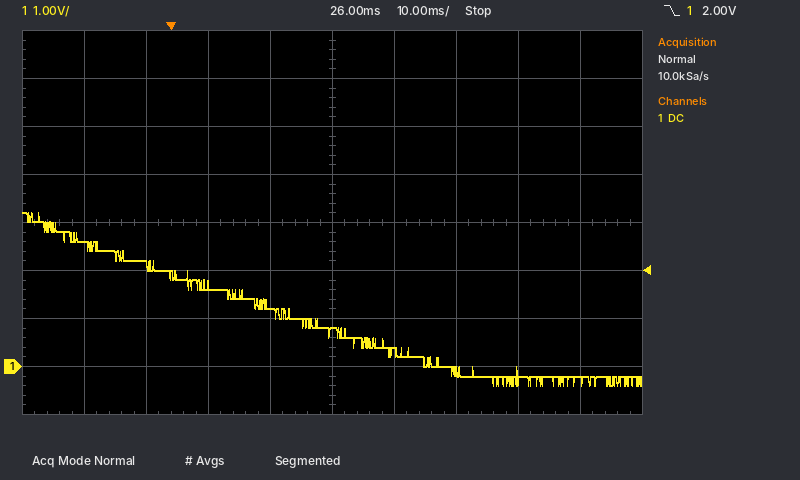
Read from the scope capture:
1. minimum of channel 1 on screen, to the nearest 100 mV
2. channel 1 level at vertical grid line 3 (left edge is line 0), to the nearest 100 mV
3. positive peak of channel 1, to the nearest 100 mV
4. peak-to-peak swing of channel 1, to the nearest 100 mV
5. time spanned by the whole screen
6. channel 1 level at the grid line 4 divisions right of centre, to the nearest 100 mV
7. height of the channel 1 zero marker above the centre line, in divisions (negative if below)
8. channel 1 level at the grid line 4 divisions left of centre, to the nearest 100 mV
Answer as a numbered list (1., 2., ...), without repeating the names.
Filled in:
1. -400 mV
2. 1.7 V
3. 3.2 V
4. 3.6 V
5. 100 ms
6. -300 mV
7. -3.0 div
8. 2.6 V
